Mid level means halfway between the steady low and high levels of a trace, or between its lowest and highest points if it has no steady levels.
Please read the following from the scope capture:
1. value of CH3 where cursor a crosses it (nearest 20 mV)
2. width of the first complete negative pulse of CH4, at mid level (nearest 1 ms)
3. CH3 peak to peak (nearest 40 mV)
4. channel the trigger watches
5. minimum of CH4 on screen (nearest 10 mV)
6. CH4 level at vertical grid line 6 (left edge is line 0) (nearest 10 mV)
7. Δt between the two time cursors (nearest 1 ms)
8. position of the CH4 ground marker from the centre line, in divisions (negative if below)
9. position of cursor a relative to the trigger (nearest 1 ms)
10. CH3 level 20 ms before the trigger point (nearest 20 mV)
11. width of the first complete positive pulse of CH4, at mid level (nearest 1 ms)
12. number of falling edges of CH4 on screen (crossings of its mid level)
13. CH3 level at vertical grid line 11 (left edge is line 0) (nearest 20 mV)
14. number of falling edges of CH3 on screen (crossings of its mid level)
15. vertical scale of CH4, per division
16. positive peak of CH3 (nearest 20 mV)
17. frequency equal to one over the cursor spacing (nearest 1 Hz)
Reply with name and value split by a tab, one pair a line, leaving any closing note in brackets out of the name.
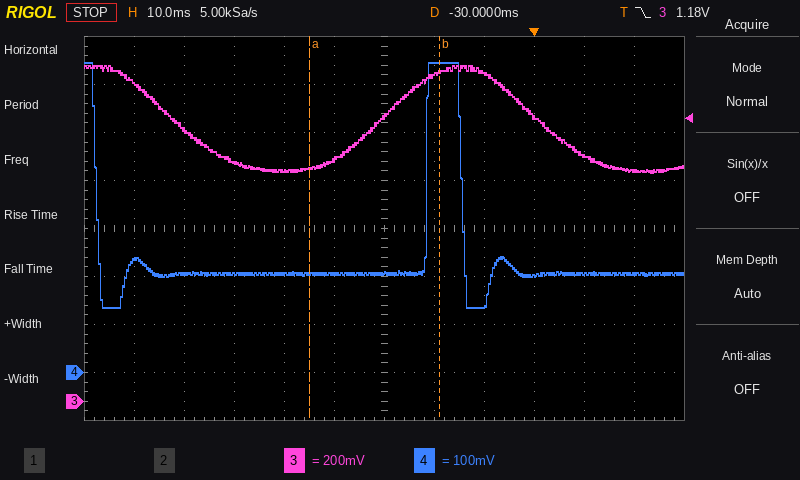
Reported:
value of CH3 where cursor a crosses it	980 mV
width of the first complete negative pulse of CH4, at mid level	66 ms
CH3 peak to peak	440 mV
channel the trigger watches	CH3
minimum of CH4 on screen	140 mV
CH4 level at vertical grid line 6 (left edge is line 0)	210 mV
Δt between the two time cursors	26 ms
position of the CH4 ground marker from the centre line, in divisions	-3.0 div
position of cursor a relative to the trigger	-45 ms
CH3 level 20 ms before the trigger point	1.36 V
width of the first complete positive pulse of CH4, at mid level	7 ms
number of falling edges of CH4 on screen	2
CH3 level at vertical grid line 11 (left edge is line 0)	960 mV
number of falling edges of CH3 on screen	2
vertical scale of CH4, per division	100 mV
positive peak of CH3	1.40 V
frequency equal to one over the cursor spacing	38 Hz
